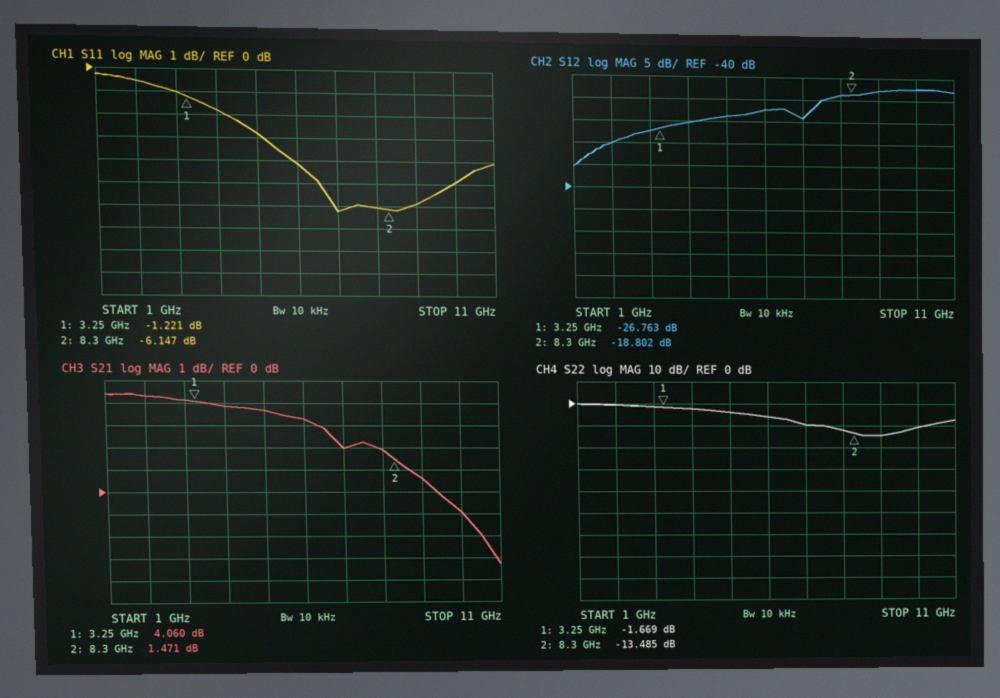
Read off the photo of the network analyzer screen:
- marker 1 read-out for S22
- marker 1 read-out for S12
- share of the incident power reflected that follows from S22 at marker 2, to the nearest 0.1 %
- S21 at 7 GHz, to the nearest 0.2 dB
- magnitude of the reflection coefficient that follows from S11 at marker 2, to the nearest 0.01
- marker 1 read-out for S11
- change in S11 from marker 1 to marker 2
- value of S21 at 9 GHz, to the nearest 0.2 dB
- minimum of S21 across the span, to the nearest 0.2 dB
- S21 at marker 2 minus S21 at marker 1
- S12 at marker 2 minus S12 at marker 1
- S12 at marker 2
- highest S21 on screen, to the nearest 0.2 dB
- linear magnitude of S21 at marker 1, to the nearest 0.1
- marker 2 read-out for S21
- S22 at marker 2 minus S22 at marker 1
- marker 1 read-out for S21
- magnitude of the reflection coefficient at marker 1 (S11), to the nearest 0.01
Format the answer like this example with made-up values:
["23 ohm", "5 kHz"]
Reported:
["-1.669 dB", "-26.763 dB", "4.5 %", "2.0 dB", "0.49", "-1.221 dB", "-4.926 dB", "0.6 dB", "-3.2 dB", "-2.589 dB", "7.961 dB", "-18.802 dB", "4.4 dB", "1.6", "1.471 dB", "-11.816 dB", "4.060 dB", "0.87"]
